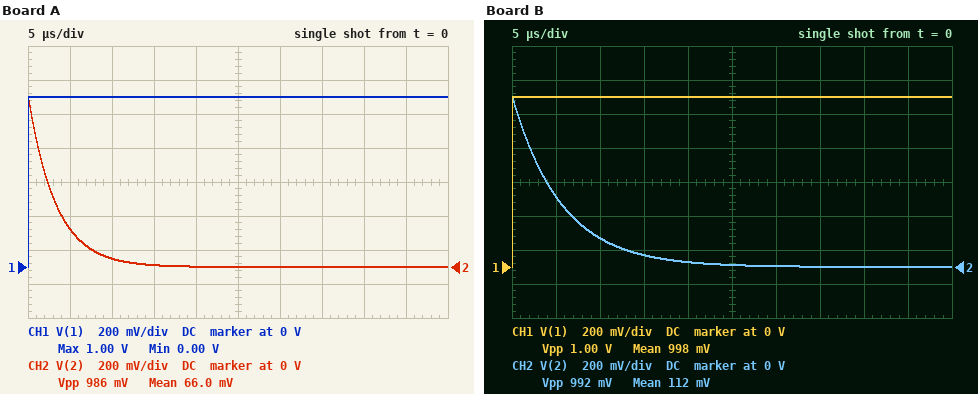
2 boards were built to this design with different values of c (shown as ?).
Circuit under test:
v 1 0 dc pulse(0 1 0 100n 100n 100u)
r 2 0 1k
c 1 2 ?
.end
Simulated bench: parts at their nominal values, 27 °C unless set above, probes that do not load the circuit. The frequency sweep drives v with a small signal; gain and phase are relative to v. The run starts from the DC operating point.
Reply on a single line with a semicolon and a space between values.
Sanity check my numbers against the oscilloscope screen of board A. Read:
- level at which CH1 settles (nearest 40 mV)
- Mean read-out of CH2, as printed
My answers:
1.00 V; 66.0 mV
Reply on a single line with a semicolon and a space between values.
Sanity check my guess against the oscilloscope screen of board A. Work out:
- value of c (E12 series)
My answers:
3.3 nF
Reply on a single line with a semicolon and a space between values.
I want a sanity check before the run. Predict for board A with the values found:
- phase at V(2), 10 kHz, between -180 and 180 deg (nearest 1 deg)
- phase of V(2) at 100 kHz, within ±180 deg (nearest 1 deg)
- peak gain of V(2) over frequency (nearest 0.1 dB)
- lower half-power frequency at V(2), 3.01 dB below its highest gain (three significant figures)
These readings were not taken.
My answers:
78 deg; 26 deg; 0 dB; 48.2 kHz
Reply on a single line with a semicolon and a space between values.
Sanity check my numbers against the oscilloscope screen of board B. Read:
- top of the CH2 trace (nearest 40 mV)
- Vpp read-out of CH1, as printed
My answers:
1.00 V; 1.00 V
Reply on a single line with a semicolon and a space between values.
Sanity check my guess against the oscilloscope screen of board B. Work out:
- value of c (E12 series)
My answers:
5.6 nF
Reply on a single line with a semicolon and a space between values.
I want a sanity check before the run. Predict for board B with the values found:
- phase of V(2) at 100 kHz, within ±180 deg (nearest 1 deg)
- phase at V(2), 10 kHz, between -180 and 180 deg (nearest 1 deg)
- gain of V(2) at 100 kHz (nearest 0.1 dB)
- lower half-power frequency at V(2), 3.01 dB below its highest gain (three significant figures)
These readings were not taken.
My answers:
16 deg; 71 deg; -0.3 dB; 28.4 kHz
